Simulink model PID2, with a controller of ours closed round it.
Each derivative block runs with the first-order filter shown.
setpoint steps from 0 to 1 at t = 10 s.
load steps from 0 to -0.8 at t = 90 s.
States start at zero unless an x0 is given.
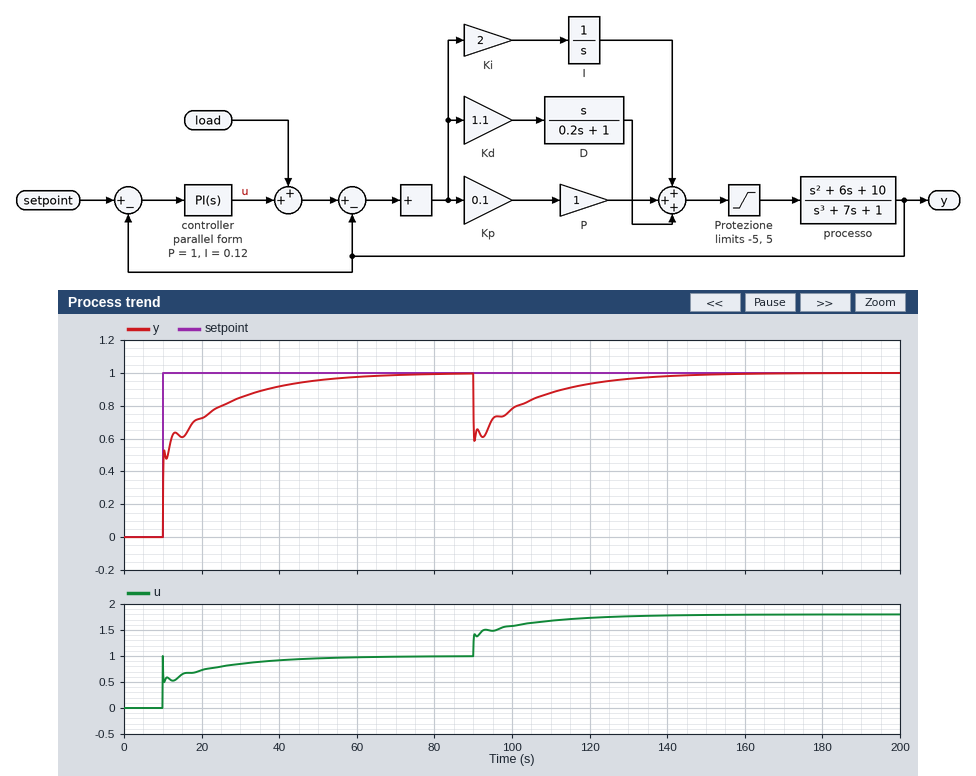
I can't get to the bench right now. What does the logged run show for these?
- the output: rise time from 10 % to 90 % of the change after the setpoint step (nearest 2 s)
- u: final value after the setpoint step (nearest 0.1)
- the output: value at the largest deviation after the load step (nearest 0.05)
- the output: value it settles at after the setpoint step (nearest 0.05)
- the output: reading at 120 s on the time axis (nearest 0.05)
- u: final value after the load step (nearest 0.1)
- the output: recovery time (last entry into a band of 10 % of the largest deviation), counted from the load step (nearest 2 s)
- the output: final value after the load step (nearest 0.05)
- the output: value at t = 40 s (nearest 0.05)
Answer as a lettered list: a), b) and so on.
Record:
a) 26 s
b) 1.0
c) 0.60
d) 1.00
e) 0.95
f) 1.8
g) 38 s
h) 1.00
i) 0.90
